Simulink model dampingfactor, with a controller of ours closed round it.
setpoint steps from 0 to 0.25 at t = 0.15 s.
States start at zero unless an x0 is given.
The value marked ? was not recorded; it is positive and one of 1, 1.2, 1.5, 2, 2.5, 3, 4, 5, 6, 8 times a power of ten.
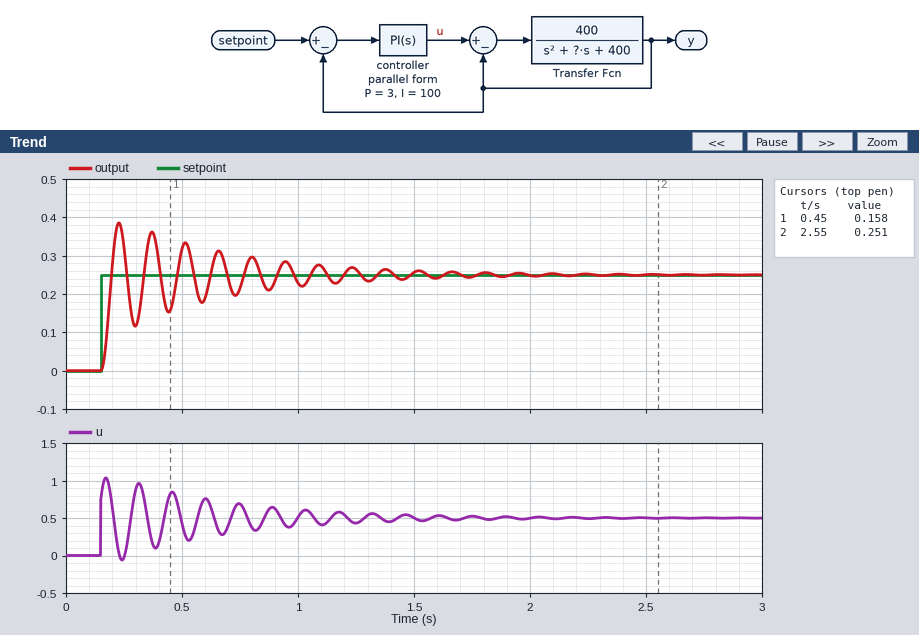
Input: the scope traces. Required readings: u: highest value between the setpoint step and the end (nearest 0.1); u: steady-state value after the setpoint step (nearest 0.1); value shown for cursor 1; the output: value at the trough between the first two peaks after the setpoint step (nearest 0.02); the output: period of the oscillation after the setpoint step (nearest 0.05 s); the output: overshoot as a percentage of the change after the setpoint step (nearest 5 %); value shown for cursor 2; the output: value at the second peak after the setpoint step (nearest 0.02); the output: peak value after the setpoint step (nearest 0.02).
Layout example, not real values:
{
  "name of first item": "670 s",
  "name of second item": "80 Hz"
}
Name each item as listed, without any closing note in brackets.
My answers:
{
  "u: highest value between the setpoint step and the end": "1.0",
  "u: steady-state value after the setpoint step": "0.5",
  "value shown for cursor 1": "0.158",
  "the output: value at the trough between the first two peaks after the setpoint step": "0.12",
  "the output: period of the oscillation after the setpoint step": "0.15 s",
  "the output: overshoot as a percentage of the change after the setpoint step": "55 %",
  "value shown for cursor 2": "0.251",
  "the output: value at the second peak after the setpoint step": "0.36",
  "the output: peak value after the setpoint step": "0.38"
}
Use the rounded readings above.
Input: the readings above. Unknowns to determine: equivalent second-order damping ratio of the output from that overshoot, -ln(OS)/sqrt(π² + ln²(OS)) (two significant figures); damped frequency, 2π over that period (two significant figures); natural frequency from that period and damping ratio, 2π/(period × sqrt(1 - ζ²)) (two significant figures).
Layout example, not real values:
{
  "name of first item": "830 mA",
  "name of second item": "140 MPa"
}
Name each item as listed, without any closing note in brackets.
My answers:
{
  "equivalent second-order damping ratio of the output from that overshoot, -ln(OS)/sqrt(π² + ln²(OS))": "0.19",
  "damped frequency, 2π over that period": "42 rad/s",
  "natural frequency from that period and damping ratio, 2π/(period × sqrt(1 - ζ²))": "43 rad/s"
}
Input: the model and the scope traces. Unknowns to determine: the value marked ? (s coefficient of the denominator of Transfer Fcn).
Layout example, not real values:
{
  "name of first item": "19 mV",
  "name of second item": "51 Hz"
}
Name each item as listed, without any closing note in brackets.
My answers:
{
  "the value marked ?": "25"
}
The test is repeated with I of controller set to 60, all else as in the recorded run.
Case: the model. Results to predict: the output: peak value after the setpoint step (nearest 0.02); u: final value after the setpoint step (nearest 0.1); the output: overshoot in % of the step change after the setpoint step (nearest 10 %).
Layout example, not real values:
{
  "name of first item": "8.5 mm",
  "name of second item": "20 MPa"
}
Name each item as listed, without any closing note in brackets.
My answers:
{
  "the output: peak value after the setpoint step": "0.32",
  "u: final value after the setpoint step": "0.5",
  "the output: overshoot in % of the step change after the setpoint step": "30 %"
}
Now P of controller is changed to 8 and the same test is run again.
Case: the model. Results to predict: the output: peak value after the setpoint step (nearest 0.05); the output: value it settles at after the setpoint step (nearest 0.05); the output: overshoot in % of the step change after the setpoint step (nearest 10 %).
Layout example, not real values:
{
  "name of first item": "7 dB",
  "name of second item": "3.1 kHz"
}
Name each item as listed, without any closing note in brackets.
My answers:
{
  "the output: peak value after the setpoint step": "0.35",
  "the output: value it settles at after the setpoint step": "0.25",
  "the output: overshoot in % of the step change after the setpoint step": "50 %"
}
